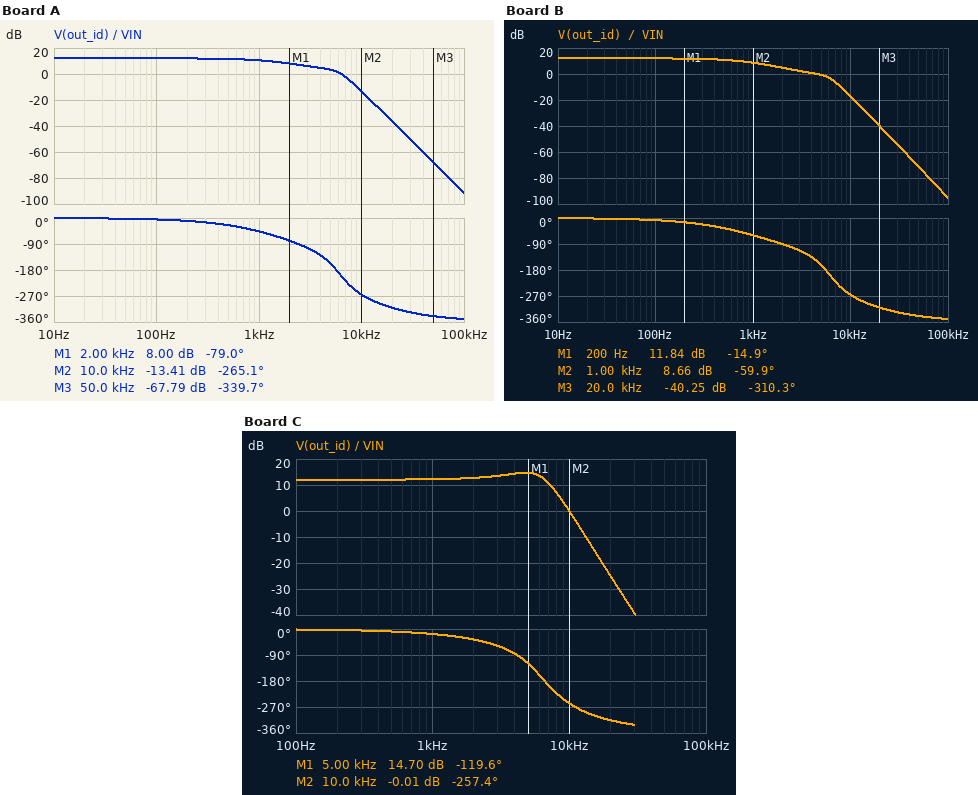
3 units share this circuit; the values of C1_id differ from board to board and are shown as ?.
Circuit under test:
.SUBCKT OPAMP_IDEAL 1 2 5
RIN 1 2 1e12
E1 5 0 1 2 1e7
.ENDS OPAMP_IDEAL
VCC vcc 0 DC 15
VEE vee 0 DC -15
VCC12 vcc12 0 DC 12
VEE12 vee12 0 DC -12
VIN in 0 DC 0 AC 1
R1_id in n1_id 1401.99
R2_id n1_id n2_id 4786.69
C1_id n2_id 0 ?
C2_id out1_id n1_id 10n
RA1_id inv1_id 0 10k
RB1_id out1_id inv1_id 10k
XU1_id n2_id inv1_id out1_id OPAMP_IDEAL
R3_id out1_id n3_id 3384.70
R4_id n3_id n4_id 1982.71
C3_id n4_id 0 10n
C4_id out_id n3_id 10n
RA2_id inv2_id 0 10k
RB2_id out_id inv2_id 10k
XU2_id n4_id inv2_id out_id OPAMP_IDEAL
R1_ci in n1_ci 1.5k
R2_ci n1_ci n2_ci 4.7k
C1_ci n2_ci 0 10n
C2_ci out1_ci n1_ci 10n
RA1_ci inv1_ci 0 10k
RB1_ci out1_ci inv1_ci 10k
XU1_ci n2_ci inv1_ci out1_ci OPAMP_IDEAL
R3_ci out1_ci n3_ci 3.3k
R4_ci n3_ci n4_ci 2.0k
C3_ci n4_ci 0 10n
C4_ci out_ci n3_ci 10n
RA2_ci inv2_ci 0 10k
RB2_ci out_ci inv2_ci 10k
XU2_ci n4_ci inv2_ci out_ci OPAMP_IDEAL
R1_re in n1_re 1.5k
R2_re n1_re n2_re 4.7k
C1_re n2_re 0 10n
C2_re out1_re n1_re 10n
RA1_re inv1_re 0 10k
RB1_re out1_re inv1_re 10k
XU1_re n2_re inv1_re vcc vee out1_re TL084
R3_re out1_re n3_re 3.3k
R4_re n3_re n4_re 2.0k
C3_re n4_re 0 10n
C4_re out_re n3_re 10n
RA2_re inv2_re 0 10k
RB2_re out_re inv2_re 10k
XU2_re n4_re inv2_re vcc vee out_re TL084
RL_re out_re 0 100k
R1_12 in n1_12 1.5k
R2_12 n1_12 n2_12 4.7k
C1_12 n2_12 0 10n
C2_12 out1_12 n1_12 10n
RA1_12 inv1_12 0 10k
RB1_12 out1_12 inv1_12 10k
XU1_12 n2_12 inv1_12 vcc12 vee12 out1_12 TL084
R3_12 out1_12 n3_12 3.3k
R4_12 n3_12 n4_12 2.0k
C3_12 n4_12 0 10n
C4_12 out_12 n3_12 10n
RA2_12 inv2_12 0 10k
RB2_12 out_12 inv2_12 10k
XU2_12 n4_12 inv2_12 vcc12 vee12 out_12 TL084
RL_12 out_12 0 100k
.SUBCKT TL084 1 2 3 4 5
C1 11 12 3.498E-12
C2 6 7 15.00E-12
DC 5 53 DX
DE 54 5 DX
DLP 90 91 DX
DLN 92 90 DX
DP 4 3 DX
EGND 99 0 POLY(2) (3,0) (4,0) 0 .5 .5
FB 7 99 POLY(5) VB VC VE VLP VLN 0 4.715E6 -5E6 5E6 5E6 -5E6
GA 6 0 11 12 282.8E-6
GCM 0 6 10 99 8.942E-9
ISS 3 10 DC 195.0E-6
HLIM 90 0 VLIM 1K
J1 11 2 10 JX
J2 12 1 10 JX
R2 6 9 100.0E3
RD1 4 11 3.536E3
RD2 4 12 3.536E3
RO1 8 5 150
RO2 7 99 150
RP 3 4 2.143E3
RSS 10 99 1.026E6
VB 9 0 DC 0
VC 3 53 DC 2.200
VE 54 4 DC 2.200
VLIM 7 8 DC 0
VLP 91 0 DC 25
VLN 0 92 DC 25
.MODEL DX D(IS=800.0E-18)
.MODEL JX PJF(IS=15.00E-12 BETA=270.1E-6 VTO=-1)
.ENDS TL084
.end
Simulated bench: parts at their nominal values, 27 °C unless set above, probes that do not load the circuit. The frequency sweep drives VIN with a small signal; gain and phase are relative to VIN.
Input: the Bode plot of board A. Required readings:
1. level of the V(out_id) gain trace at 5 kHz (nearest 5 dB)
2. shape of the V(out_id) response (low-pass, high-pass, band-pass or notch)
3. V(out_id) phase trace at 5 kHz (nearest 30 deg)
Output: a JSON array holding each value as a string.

["5 dB", "low-pass", "-150 deg"]
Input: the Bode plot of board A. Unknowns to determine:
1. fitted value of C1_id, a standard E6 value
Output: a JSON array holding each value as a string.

["22 nF"]
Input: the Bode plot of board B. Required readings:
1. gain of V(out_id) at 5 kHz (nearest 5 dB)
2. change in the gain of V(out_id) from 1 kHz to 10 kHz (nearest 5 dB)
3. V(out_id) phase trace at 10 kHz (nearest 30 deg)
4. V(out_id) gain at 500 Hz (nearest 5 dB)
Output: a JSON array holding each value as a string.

["0 dB", "-25 dB", "-270 deg", "10 dB"]
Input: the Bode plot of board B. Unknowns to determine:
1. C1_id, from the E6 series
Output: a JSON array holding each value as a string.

["33 nF"]
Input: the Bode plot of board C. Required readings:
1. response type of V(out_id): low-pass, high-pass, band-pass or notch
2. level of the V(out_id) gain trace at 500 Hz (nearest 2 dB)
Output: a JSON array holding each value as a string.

["low-pass", "12 dB"]
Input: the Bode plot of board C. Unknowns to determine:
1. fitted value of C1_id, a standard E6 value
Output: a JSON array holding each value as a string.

["6.8 nF"]
